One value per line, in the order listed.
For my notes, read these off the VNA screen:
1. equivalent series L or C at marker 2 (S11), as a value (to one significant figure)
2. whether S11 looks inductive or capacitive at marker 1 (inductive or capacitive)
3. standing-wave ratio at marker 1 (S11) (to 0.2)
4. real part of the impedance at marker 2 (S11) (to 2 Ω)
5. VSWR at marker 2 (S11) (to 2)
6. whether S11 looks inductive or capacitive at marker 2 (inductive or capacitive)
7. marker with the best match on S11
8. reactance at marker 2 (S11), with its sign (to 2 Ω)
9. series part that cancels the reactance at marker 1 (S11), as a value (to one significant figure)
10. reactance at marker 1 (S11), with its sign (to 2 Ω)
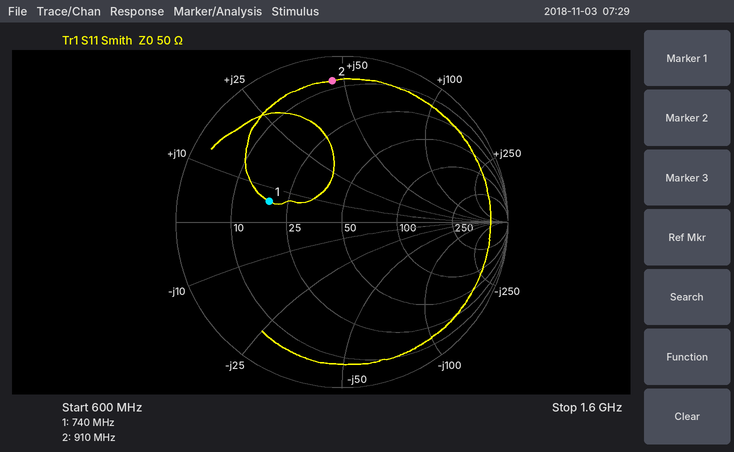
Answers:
8 nH
inductive
2.6
8 Ω
12
inductive
marker 1
+46 Ω
40 pF
+6 Ω
